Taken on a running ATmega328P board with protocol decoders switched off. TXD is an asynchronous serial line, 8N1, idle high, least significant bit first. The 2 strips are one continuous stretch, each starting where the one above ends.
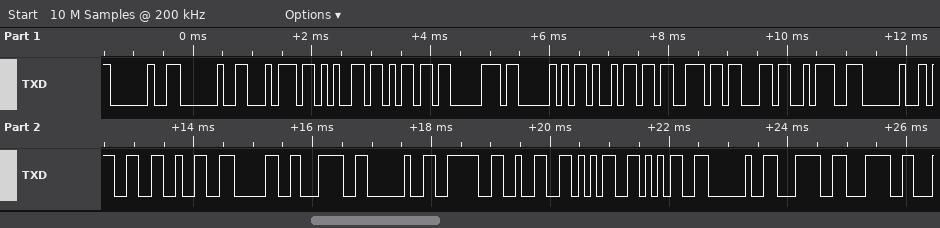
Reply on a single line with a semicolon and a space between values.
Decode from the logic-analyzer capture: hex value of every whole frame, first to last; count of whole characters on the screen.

20 20 74 65 6D 70 50 69 73 63 3A 20 33 32 30 3C 20 3E 32 35 35 20 3C 3C; 24
